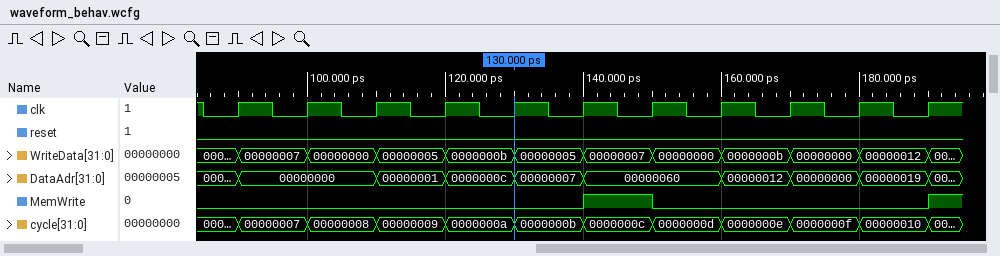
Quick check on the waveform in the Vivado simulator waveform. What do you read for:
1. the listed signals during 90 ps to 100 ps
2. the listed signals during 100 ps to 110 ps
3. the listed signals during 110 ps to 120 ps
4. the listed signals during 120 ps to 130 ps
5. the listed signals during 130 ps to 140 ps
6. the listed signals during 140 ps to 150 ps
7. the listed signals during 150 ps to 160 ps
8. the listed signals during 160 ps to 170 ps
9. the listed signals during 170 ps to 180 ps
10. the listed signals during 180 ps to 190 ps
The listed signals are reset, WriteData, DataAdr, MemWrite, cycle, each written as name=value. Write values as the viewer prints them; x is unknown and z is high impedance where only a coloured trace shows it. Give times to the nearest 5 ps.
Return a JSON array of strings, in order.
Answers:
["reset=0, WriteData=00000007, DataAdr=00000000, MemWrite=0, cycle=00000007", "reset=0, WriteData=00000000, DataAdr=00000000, MemWrite=0, cycle=00000008", "reset=0, WriteData=00000005, DataAdr=00000001, MemWrite=0, cycle=00000009", "reset=0, WriteData=0000000b, DataAdr=0000000c, MemWrite=0, cycle=0000000a", "reset=0, WriteData=00000005, DataAdr=00000007, MemWrite=0, cycle=0000000b", "reset=0, WriteData=00000007, DataAdr=00000060, MemWrite=1, cycle=0000000c", "reset=0, WriteData=00000000, DataAdr=00000060, MemWrite=0, cycle=0000000d", "reset=0, WriteData=0000000b, DataAdr=00000012, MemWrite=0, cycle=0000000e", "reset=0, WriteData=00000000, DataAdr=00000000, MemWrite=0, cycle=0000000f", "reset=0, WriteData=00000012, DataAdr=00000019, MemWrite=0, cycle=00000010"]
